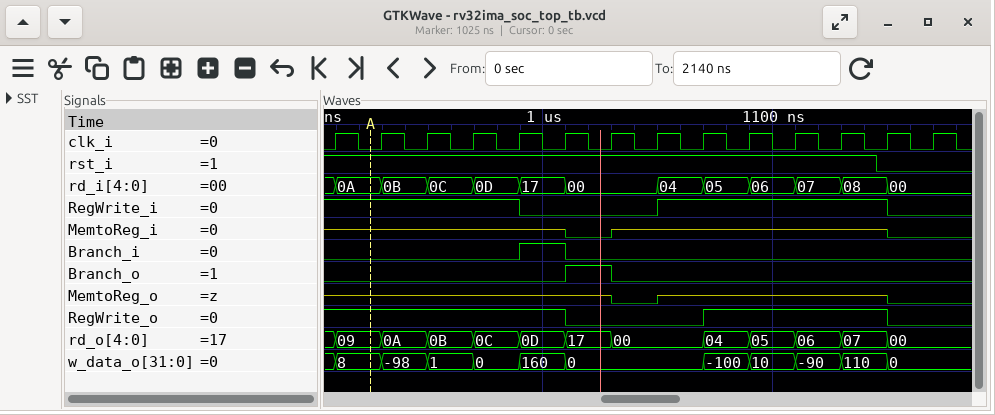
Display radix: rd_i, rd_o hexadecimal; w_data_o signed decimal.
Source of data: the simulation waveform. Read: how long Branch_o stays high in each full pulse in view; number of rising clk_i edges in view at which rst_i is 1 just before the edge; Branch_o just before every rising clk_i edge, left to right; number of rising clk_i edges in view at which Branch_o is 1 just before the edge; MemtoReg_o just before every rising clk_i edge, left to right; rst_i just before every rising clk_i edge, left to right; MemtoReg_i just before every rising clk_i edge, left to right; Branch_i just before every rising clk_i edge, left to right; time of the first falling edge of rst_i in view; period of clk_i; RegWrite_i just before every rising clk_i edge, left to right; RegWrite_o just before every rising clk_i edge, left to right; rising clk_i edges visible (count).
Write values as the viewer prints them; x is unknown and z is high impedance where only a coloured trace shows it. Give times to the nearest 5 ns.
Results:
20 ns
12
0 0 0 0 0 0 1 0 0 0 0 0 0 0
1
z z z z z z z 0 z z z z z 0
1 1 1 1 1 1 1 1 1 1 1 1 0 0
z z z z z z 0 z z z z z z 0
0 0 0 0 0 1 0 0 0 0 0 0 0 0
1145 ns
20 ns
1 1 1 1 1 0 0 0 1 1 1 1 1 0
1 1 1 1 1 1 0 0 0 1 1 1 1 0
14
